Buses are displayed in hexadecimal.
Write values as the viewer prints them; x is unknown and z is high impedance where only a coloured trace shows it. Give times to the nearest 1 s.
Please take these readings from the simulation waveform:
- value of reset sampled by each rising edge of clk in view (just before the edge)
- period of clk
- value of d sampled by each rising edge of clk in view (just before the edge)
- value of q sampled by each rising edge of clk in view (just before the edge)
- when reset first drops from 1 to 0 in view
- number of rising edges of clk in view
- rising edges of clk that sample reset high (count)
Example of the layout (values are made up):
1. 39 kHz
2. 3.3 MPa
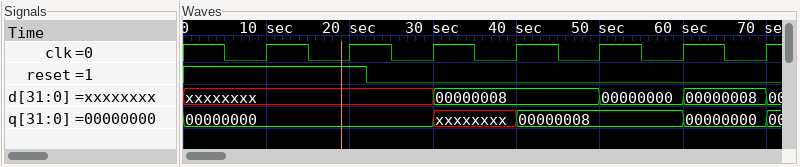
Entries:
1. 1 1 0 0 0 0 0
2. 10 s
3. xxxxxxxx, xxxxxxxx, xxxxxxxx, 00000008, 00000008, 00000000, 00000008
4. 00000000, 00000000, 00000000, xxxxxxxx, 00000008, 00000008, 00000000
5. 22 s
6. 7
7. 2
